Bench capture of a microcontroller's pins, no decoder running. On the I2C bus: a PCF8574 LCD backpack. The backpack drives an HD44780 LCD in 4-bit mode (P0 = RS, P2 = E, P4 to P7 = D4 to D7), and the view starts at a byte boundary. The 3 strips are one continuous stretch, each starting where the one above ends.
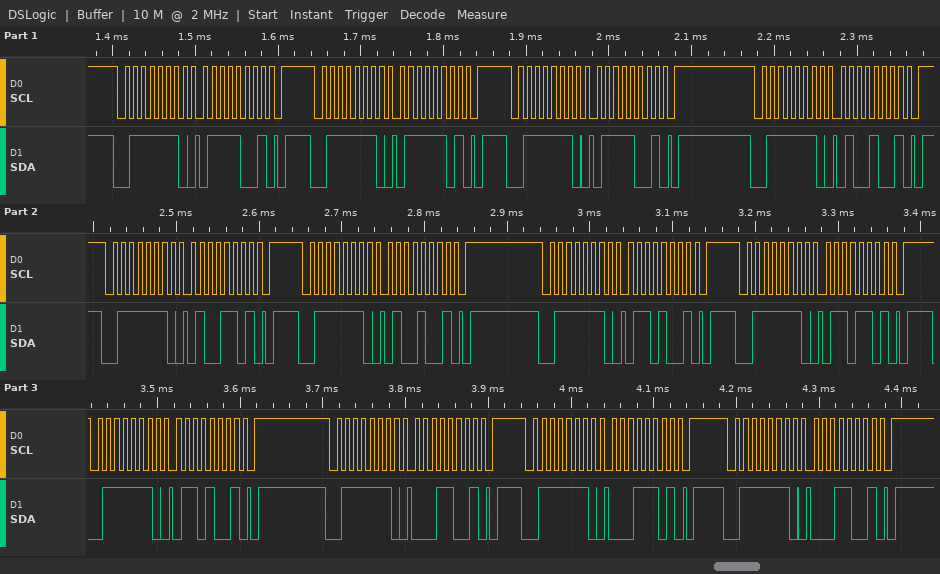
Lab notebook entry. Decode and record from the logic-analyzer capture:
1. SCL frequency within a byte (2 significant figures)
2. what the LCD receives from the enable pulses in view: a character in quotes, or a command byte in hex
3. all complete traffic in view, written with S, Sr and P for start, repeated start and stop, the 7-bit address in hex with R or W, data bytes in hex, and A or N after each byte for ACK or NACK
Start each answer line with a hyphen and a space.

- 100 kHz
- 't' 'a'
- S 3FW A 79 A P S 3FW A 7D A P S 3FW A 79 A P S 3FW A 49 A P S 3FW A 4D A P S 3FW A 49 A P S 3FW A 69 A P S 3FW A 6D A P S 3FW A 69 A P S 3FW A 19 A P S 3FW A 1D A P S 3FW A 19 A P
